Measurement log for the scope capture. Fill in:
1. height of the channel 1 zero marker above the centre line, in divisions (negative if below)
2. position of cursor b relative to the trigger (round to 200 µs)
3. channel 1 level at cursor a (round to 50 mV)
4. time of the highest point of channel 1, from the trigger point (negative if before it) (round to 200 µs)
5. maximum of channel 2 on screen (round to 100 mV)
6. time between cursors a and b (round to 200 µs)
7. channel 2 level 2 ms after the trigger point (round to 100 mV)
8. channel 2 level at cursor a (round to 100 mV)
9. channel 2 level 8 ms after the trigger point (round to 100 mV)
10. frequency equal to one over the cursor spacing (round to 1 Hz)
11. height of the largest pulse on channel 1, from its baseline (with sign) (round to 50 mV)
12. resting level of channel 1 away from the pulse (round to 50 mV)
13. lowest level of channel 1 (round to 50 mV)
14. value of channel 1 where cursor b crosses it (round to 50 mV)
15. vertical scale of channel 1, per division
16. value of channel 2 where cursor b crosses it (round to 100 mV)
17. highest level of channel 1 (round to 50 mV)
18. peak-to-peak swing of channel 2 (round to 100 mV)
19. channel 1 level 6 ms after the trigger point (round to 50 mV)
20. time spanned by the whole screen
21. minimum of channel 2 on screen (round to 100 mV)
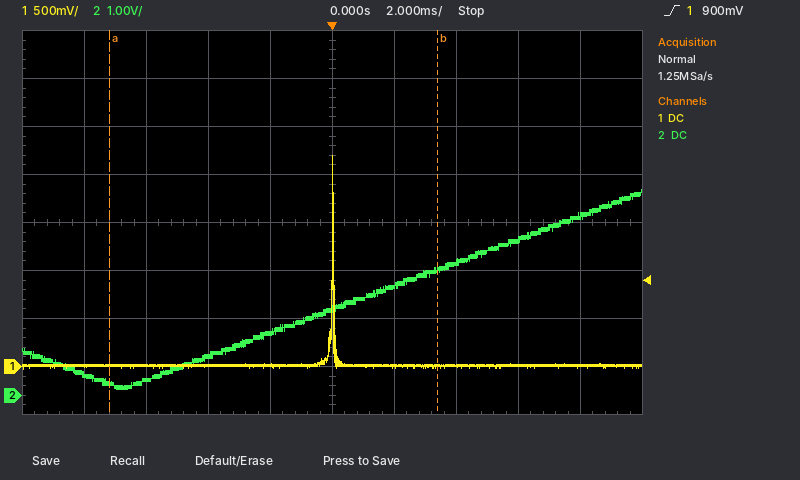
-3.0 div
+3.4 ms
0 mV
0.0 ms
4.3 V
10.6 ms
2.3 V
200 mV
3.7 V
94 Hz
+2.20 V
0 mV
-50 mV
0 mV
500 mV
2.6 V
2.20 V
4.2 V
0 mV
20 ms
100 mV
